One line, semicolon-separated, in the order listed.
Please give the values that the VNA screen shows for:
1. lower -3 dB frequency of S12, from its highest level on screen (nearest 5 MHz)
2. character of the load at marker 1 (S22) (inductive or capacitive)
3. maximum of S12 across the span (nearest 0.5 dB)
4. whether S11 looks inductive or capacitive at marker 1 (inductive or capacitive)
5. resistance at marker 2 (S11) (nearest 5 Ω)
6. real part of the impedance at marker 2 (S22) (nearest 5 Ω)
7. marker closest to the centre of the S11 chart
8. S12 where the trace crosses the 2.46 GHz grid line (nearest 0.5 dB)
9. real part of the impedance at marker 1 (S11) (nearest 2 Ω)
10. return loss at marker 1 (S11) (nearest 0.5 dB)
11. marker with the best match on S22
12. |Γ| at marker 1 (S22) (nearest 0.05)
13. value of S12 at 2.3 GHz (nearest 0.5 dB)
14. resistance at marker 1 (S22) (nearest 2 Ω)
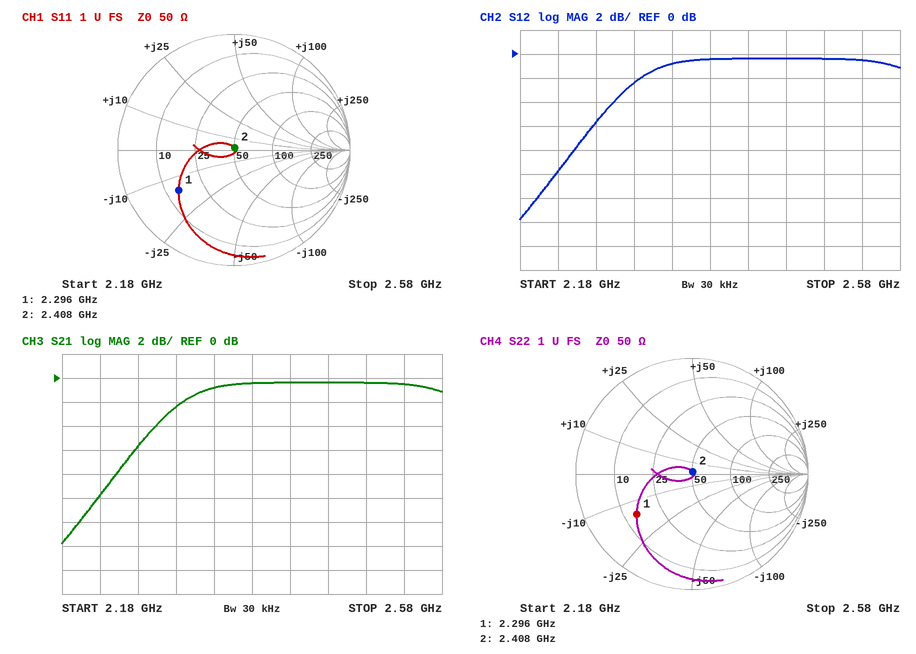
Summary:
2.285 GHz; capacitive; -0.5 dB; capacitive; 50 Ω; 50 Ω; marker 2; -0.5 dB; 14 Ω; 4.5 dB; marker 2; 0.60; -2.5 dB; 14 Ω
